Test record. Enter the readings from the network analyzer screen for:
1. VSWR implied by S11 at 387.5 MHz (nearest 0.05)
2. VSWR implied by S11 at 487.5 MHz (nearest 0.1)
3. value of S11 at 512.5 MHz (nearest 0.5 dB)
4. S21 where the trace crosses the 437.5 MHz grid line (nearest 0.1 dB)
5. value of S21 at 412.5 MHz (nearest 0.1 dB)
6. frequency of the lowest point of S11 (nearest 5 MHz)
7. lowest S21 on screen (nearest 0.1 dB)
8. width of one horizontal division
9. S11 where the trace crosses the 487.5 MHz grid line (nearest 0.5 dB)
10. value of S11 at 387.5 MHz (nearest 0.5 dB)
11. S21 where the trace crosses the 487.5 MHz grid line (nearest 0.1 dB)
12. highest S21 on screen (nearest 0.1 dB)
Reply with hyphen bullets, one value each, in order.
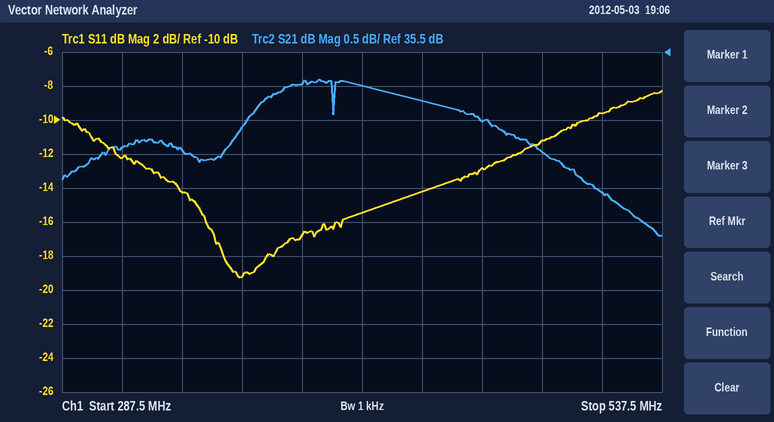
- 1.35
- 1.8
- -9.5 dB
- 34.8 dB
- 35.0 dB
- 360 MHz
- 32.8 dB
- 25 MHz
- -11.0 dB
- -17.0 dB
- 34.0 dB
- 35.1 dB
